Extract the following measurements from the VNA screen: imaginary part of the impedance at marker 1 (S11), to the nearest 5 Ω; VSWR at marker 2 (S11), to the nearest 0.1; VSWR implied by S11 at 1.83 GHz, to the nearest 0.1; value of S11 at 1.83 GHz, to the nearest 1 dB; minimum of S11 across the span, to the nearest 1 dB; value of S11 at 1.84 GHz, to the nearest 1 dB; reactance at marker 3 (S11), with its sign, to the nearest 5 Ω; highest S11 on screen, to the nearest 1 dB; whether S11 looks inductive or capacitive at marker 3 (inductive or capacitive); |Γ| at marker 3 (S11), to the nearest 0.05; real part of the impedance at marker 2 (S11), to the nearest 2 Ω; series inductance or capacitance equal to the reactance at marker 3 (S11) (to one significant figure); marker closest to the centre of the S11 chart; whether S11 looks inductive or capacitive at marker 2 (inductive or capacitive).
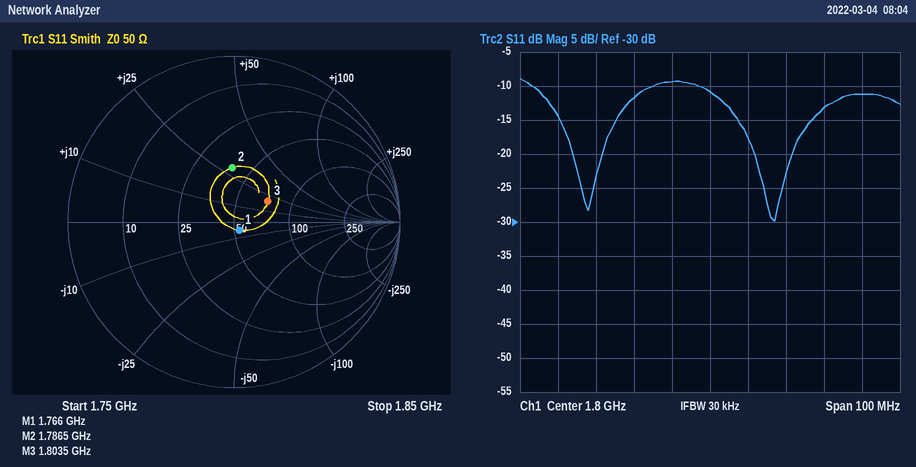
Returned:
-5 Ω
2.0
1.6
-13 dB
-30 dB
-11 dB
+20 Ω
-9 dB
inductive
0.25
40 Ω
2 nH
marker 1
inductive
